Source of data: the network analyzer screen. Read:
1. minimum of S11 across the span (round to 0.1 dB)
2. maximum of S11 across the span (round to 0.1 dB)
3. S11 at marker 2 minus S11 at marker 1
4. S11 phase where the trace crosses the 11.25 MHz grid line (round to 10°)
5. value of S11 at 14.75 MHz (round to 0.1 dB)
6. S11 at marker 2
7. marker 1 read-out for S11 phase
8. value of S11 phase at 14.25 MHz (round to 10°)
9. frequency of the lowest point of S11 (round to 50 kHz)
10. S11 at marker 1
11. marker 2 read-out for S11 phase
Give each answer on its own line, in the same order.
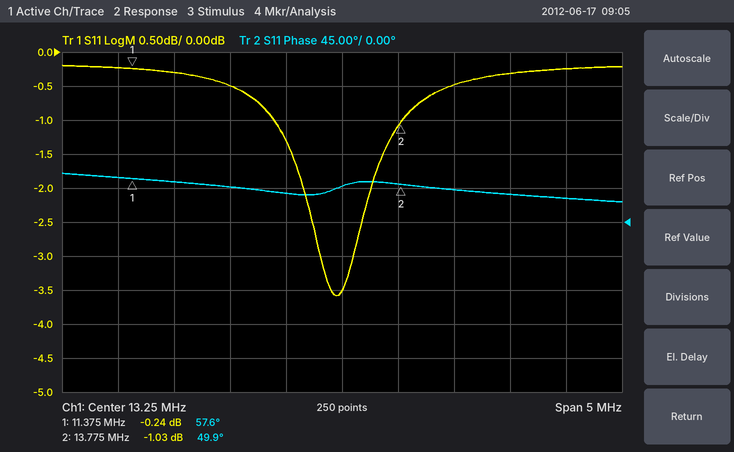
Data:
-3.6 dB
-0.2 dB
-0.79 dB
60°
-0.3 dB
-1.03 dB
57.6°
40°
13.20 MHz
-0.24 dB
49.9°
